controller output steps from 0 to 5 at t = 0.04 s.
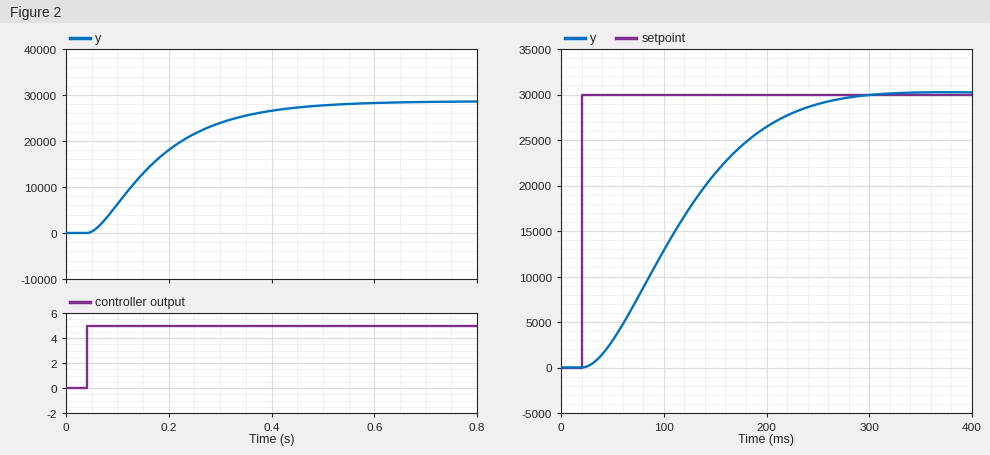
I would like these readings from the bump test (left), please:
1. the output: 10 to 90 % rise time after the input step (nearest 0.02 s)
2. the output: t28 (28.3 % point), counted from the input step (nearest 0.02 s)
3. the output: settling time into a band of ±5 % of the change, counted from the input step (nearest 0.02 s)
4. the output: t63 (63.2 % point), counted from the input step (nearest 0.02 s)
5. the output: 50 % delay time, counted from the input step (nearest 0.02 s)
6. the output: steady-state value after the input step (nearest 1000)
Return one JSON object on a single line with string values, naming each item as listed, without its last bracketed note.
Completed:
{"the output: 10 to 90 % rise time after the input step": "0.28 s", "the output: t28 (28.3 % point), counted from the input step": "0.08 s", "the output: settling time into a band of ±5 % of the change, counted from the input step": "0.40 s", "the output: t63 (63.2 % point), counted from the input step": "0.16 s", "the output: 50 % delay time, counted from the input step": "0.12 s", "the output: steady-state value after the input step": "29000"}
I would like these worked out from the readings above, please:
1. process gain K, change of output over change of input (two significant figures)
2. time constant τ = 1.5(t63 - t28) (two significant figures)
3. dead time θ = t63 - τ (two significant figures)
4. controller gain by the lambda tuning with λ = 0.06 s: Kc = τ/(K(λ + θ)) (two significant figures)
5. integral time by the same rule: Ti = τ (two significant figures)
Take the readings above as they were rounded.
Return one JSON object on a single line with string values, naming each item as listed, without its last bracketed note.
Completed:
{"process gain K, change of output over change of input": "5800", "time constant τ = 1.5(t63 - t28)": "0.12 s", "dead time θ = t63 - τ": "0.040 s", "controller gain by the lambda tuning with λ = 0.06 s: Kc = τ/(K(λ + θ))": "0.00021", "integral time by the same rule: Ti = τ": "0.12 s"}
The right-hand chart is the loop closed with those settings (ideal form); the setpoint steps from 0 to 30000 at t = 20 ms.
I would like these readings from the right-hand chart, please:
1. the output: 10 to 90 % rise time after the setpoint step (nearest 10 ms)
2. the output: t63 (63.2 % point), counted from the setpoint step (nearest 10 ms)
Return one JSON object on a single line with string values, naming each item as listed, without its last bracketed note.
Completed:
{"the output: 10 to 90 % rise time after the setpoint step": "160 ms", "the output: t63 (63.2 % point), counted from the setpoint step": "110 ms"}
